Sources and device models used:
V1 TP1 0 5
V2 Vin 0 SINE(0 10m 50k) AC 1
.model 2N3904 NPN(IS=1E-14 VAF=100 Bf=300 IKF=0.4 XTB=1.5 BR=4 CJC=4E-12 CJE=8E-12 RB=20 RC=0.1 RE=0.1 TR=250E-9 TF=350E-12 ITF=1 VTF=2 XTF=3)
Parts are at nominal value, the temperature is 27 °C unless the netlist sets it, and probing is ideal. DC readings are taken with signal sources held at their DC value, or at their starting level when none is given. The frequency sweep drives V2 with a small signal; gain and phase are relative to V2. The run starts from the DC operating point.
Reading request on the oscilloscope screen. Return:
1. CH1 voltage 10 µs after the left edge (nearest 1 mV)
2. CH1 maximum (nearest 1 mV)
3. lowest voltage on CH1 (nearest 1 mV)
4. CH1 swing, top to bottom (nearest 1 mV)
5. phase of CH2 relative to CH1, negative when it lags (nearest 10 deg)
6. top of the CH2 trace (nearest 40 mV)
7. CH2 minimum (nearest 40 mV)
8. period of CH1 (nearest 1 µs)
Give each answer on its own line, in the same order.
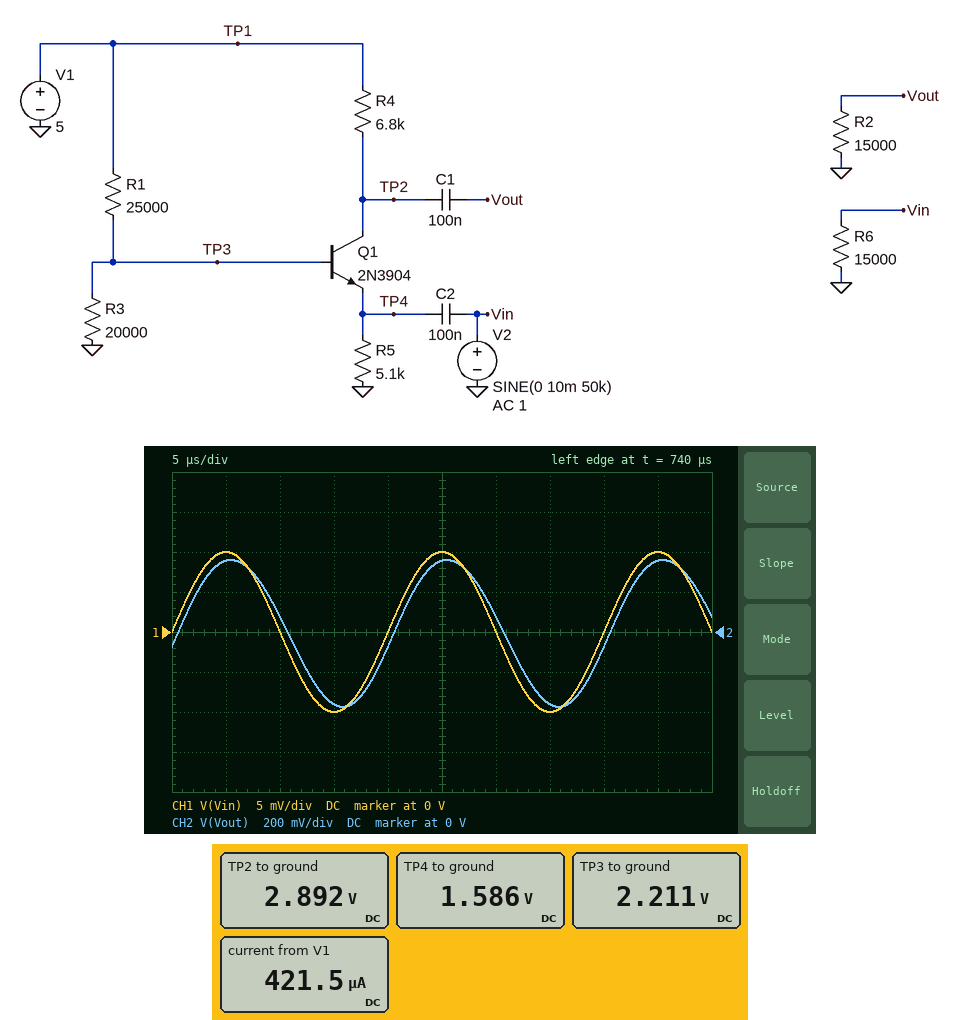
0 V
10 mV
-10 mV
20 mV
-10 deg
360 mV
-360 mV
20 µs
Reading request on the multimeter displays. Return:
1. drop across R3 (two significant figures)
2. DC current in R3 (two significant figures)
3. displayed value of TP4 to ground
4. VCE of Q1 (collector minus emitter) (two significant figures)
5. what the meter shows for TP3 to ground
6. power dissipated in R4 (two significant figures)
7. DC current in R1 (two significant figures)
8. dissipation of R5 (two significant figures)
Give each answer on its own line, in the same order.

2.2 V
110 µA
1.586 V
1.3 V
2.211 V
650 µW
110 µA
490 µW
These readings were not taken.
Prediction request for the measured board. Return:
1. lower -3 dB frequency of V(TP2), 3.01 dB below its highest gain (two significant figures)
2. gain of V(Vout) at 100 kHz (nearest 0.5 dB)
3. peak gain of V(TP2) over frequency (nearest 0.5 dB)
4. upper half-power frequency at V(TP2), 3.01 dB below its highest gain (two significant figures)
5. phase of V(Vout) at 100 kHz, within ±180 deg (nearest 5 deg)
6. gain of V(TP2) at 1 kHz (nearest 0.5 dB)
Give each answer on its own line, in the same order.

12 kHz
29.5 dB
31.5 dB
120 kHz
-40 deg
9.0 dB
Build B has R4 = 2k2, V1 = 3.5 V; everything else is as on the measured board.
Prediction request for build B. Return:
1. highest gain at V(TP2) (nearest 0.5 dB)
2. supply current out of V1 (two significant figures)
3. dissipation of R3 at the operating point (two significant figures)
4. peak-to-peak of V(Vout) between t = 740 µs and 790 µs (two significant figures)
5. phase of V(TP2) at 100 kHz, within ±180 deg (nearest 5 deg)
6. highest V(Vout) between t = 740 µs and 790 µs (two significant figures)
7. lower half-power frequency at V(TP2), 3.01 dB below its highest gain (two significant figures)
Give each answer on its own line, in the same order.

20.5 dB
260 µA
120 µW
210 mV
-10 deg
100 mV
9.0 kHz
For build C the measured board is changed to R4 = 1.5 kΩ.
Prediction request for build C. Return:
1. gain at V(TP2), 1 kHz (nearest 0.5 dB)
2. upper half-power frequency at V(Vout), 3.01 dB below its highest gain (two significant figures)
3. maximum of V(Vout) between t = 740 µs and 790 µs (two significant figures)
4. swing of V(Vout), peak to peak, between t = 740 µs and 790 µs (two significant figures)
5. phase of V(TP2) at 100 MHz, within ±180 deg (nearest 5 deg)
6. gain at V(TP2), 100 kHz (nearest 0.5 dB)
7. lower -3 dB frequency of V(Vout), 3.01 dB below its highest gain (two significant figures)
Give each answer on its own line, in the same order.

-1.5 dB
360 kHz
110 mV
220 mV
10 deg
21.0 dB
13 kHz
